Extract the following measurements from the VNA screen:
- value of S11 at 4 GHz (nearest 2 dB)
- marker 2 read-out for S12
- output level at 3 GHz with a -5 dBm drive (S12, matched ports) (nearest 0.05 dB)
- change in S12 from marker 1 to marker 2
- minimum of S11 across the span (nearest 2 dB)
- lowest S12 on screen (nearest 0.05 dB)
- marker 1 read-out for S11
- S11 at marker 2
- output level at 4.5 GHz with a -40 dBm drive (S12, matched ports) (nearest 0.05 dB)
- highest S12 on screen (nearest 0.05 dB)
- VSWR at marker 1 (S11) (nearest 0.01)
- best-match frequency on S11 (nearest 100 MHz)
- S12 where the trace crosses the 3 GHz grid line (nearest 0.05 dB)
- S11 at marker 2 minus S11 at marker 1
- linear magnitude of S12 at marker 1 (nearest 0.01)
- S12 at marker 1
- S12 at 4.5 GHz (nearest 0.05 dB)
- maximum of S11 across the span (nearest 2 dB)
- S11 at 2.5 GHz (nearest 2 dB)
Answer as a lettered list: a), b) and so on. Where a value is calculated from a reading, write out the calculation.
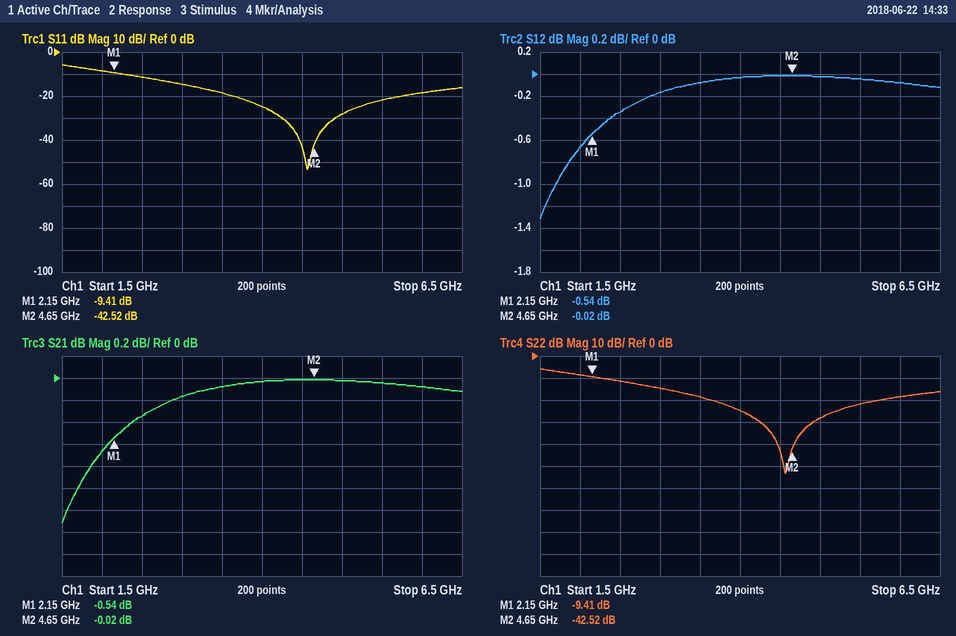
a) -24 dB
b) -0.02 dB
c) -5 dBm + (-0.15 dB) = -5.15 dBm
d) -0.02 − (-0.54) = 0.52 dB
e) -54 dB
f) -1.30 dB
g) -9.41 dB
h) -42.52 dB
i) -40 dBm + (0.00 dB) = -40.00 dBm
j) 0.00 dB
k) (1 + 0.3385)/(1 − 0.3385) ≈ 2.02
l) 4.6 GHz
m) -0.15 dB
n) -42.52 − (-9.41) = -33.11 dB
o) 10^(-0.54/20) ≈ 0.94
p) -0.54 dB
q) 0.00 dB
r) -6 dB
s) -12 dB
